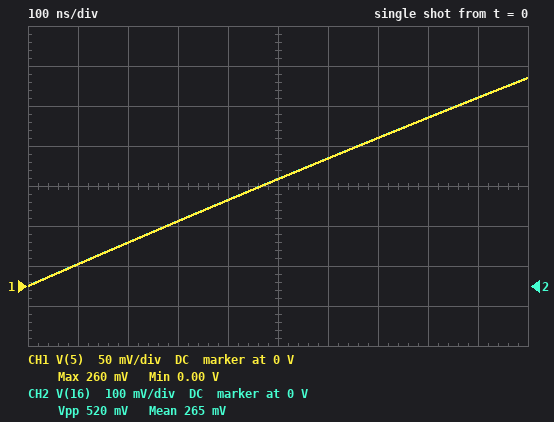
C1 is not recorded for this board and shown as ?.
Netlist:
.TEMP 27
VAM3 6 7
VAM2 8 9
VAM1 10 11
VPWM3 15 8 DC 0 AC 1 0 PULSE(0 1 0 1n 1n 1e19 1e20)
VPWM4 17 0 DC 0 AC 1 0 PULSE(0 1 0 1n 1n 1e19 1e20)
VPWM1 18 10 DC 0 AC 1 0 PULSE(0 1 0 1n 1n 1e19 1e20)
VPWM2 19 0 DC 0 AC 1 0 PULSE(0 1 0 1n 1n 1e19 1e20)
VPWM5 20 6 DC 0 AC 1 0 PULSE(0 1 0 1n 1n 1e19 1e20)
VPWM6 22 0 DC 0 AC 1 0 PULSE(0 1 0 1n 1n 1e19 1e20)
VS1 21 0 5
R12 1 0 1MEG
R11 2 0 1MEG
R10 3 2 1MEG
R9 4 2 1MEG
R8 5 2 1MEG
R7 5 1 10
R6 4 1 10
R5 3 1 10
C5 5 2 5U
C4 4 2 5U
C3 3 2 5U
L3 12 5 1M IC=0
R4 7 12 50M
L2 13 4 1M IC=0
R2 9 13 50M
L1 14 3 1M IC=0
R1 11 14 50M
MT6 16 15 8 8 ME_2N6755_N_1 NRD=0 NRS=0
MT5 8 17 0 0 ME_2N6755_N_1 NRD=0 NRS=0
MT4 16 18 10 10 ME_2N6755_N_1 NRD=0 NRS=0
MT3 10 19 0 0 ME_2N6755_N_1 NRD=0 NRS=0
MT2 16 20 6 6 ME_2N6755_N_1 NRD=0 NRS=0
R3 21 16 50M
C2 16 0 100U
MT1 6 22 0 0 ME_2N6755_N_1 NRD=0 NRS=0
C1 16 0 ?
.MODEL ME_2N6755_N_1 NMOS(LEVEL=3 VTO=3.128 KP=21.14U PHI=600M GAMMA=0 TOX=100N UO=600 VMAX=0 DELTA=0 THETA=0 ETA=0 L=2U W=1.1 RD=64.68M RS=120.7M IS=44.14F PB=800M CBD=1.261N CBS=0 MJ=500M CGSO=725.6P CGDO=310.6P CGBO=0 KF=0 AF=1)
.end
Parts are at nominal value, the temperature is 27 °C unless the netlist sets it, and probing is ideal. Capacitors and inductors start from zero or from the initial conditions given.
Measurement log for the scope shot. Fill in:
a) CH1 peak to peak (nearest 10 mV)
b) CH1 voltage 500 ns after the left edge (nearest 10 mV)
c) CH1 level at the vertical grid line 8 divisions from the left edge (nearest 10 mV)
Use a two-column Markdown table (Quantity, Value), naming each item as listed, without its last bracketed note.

| Quantity | Value |
|---|---|
| CH1 peak to peak | 260 mV |
| CH1 voltage 500 ns after the left edge | 130 mV |
| CH1 level at the vertical grid line 8 divisions from the left edge | 210 mV |
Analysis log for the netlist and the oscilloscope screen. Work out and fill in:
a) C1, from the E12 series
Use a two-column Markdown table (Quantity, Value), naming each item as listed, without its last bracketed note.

| Quantity | Value |
|---|---|
| C1, from the E12 series | 82 µF |
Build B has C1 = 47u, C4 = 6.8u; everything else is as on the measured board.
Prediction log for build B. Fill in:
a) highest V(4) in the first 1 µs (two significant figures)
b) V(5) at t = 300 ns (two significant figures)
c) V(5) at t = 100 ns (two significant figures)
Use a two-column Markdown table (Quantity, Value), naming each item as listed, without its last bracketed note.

| Quantity | Value |
|---|---|
| highest V(4) in the first 1 µs | 320 mV |
| V(5) at t = 300 ns | 100 mV |
| V(5) at t = 100 ns | 34 mV |
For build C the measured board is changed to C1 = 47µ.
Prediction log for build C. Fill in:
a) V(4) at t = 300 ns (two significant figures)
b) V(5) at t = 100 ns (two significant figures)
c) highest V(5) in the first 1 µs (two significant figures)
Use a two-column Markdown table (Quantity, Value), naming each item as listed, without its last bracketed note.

| Quantity | Value |
|---|---|
| V(4) at t = 300 ns | 100 mV |
| V(5) at t = 100 ns | 34 mV |
| highest V(5) in the first 1 µs | 320 mV |
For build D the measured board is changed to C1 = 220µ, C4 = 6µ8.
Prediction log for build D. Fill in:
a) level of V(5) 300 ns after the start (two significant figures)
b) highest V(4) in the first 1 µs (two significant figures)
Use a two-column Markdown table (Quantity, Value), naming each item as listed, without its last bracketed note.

| Quantity | Value |
|---|---|
| level of V(5) 300 ns after the start | 46 mV |
| highest V(4) in the first 1 µs | 150 mV |
